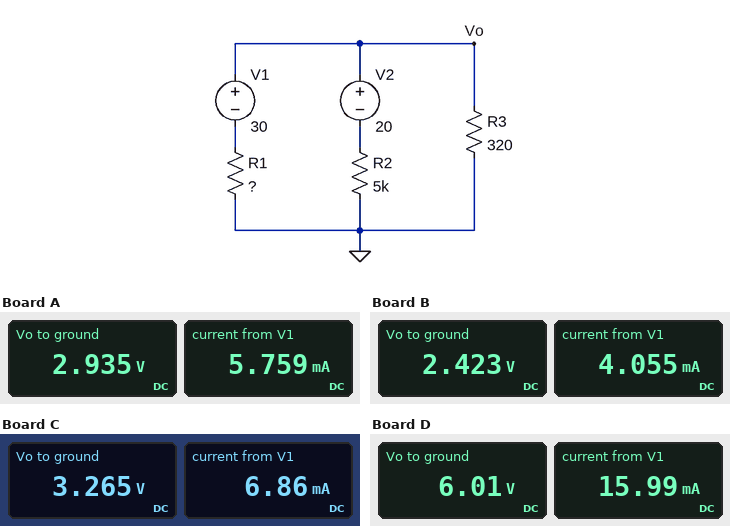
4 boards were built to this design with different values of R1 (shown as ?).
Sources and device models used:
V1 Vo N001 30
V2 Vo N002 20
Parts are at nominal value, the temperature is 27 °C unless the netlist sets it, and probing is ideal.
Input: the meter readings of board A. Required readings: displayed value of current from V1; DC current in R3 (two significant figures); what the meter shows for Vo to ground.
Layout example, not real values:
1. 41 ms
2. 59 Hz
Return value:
1. 5.759 mA
2. 9.2 mA
3. 2.935 V
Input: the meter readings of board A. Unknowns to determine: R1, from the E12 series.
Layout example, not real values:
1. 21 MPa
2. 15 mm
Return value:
1. 4.7 kΩ
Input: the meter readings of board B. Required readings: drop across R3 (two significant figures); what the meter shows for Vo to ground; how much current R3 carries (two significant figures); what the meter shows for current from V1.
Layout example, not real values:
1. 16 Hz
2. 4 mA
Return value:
1. 2.4 V
2. 2.423 V
3. 7.6 mA
4. 4.055 mA
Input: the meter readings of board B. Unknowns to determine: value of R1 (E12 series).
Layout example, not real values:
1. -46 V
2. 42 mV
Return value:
1. 6.8 kΩ
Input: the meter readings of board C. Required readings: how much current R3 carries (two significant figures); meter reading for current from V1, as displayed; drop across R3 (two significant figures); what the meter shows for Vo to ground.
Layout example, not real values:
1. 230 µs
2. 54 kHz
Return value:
1. 10 mA
2. 6.86 mA
3. 3.3 V
4. 3.265 V
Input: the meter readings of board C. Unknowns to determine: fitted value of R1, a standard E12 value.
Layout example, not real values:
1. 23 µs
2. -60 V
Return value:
1. 3.9 kΩ
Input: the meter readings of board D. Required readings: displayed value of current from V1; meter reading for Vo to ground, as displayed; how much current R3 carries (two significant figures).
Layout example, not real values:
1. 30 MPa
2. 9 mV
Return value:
1. 15.99 mA
2. 6.01 V
3. 19 mA
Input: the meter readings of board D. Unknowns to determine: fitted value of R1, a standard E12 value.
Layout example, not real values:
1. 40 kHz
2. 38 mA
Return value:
1. 1.5 kΩ
